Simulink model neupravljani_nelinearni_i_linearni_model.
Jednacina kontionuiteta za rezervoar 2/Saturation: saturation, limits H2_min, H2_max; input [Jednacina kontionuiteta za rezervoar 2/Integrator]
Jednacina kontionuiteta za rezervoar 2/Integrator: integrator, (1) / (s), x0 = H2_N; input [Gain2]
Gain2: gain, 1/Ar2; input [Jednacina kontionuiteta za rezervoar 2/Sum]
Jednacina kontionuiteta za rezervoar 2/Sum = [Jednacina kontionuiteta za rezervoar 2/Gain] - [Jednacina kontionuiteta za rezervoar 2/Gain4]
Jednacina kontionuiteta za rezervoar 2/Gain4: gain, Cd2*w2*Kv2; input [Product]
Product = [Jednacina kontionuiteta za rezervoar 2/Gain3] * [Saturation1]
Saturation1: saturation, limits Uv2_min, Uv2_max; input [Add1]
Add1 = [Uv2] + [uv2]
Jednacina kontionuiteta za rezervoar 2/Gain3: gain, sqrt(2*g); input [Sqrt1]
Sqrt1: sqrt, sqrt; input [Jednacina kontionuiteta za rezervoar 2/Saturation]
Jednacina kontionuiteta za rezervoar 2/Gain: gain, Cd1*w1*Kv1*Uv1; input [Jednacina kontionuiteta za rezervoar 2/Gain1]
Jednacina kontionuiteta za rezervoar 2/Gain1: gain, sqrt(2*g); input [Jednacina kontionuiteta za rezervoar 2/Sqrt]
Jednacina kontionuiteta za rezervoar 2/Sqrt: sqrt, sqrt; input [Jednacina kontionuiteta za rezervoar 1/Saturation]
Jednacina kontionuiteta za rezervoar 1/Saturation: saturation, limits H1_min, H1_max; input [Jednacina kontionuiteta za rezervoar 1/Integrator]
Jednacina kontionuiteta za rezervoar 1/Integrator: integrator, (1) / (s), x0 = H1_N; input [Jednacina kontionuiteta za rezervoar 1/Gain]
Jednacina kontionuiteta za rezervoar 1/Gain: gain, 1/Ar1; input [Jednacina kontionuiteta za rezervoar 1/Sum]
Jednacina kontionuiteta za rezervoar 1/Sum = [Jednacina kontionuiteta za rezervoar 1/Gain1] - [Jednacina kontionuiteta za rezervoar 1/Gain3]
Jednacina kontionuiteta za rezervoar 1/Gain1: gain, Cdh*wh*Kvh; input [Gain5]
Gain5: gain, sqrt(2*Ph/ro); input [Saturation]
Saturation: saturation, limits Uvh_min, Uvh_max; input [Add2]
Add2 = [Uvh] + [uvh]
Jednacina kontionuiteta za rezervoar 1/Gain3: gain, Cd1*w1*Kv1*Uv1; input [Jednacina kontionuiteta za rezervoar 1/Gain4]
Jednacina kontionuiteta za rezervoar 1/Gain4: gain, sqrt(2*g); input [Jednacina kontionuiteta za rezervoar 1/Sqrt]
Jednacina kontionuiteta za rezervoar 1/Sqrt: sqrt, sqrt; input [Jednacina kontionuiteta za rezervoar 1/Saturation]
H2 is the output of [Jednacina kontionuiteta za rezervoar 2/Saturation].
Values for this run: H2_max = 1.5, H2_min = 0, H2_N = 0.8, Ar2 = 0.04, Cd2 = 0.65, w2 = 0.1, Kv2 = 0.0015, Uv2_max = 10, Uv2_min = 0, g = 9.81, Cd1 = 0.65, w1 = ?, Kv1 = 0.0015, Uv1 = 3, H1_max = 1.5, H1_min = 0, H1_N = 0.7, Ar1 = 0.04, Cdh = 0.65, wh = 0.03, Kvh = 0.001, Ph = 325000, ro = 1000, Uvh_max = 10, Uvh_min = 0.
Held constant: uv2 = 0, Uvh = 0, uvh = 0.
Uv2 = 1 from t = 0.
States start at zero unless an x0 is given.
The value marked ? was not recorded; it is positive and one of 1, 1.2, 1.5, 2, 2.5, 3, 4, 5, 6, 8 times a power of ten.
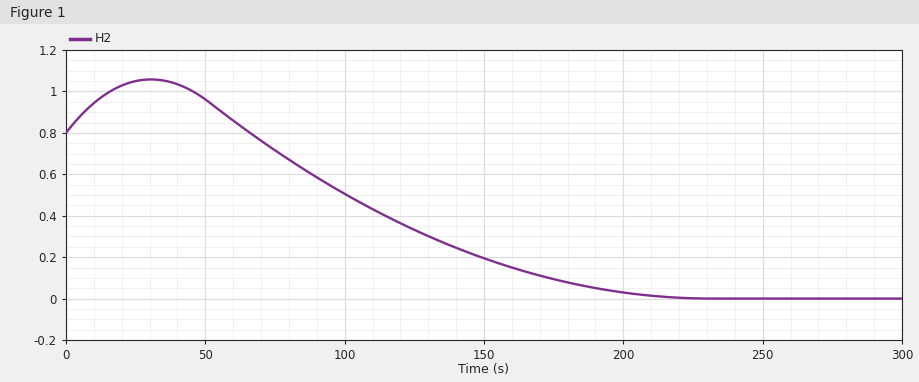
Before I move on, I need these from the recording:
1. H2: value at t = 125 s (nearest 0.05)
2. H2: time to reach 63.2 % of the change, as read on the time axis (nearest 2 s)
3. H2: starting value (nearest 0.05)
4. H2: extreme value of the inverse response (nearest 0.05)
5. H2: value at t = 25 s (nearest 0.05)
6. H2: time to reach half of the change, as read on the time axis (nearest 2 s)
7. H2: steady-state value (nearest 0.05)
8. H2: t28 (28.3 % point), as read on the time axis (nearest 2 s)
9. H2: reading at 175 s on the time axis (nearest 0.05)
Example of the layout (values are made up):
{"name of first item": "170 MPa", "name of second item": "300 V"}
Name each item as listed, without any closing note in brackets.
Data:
{"H2: value at t = 125 s": "0.35", "H2: time to reach 63.2 % of the change, as read on the time axis": "132 s", "H2: starting value": "0.80", "H2: extreme value of the inverse response": "1.05", "H2: value at t = 25 s": "1.05", "H2: time to reach half of the change, as read on the time axis": "114 s", "H2: steady-state value": "0.00", "H2: t28 (28.3 % point), as read on the time axis": "92 s", "H2: reading at 175 s on the time axis": "0.10"}
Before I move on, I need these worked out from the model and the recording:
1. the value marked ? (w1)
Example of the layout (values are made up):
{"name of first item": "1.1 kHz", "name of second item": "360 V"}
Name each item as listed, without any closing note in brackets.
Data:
{"the value marked ?": "0.1"}
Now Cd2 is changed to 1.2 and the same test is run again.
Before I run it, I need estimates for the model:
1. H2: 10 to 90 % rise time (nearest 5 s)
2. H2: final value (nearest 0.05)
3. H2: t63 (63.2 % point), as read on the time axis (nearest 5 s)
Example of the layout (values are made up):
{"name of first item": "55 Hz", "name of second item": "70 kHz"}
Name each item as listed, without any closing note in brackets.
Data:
{"H2: 10 to 90 % rise time": "60 s", "H2: final value": "0.00", "H2: t63 (63.2 % point), as read on the time axis": "75 s"}
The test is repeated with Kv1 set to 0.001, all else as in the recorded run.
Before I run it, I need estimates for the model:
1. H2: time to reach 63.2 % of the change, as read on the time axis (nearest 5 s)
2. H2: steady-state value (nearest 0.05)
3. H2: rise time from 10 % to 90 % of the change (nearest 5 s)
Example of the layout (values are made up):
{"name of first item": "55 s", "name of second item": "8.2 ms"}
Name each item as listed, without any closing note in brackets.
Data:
{"H2: time to reach 63.2 % of the change, as read on the time axis": "135 s", "H2: steady-state value": "0.00", "H2: rise time from 10 % to 90 % of the change": "105 s"}
